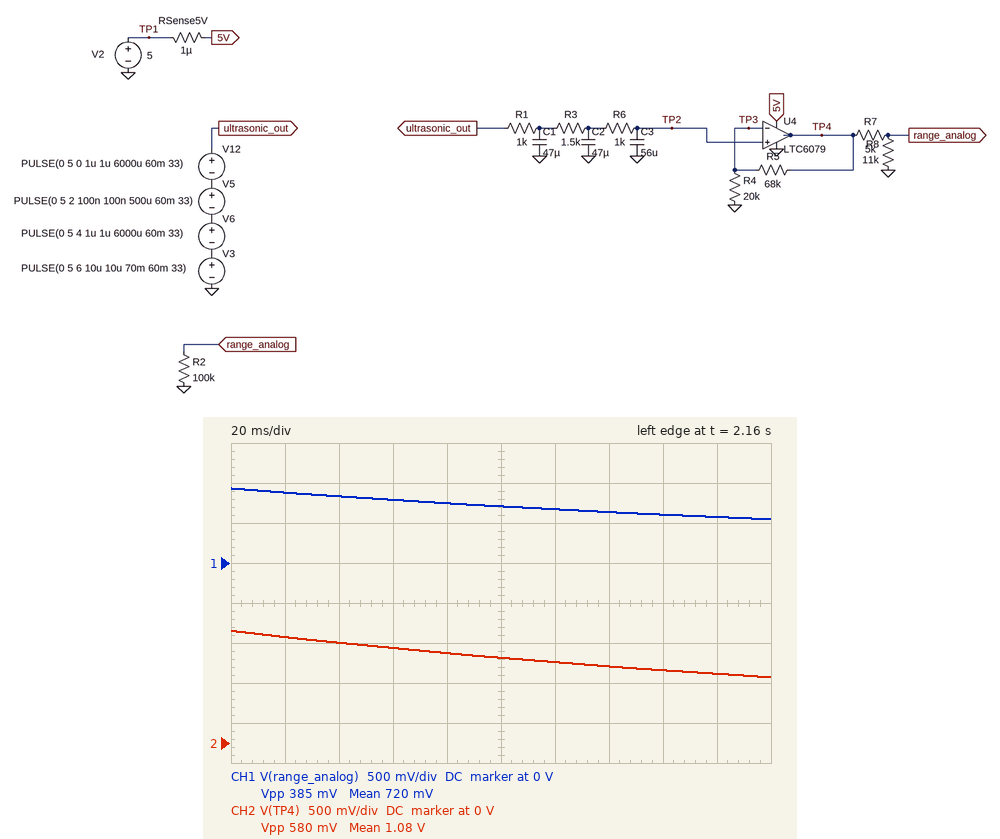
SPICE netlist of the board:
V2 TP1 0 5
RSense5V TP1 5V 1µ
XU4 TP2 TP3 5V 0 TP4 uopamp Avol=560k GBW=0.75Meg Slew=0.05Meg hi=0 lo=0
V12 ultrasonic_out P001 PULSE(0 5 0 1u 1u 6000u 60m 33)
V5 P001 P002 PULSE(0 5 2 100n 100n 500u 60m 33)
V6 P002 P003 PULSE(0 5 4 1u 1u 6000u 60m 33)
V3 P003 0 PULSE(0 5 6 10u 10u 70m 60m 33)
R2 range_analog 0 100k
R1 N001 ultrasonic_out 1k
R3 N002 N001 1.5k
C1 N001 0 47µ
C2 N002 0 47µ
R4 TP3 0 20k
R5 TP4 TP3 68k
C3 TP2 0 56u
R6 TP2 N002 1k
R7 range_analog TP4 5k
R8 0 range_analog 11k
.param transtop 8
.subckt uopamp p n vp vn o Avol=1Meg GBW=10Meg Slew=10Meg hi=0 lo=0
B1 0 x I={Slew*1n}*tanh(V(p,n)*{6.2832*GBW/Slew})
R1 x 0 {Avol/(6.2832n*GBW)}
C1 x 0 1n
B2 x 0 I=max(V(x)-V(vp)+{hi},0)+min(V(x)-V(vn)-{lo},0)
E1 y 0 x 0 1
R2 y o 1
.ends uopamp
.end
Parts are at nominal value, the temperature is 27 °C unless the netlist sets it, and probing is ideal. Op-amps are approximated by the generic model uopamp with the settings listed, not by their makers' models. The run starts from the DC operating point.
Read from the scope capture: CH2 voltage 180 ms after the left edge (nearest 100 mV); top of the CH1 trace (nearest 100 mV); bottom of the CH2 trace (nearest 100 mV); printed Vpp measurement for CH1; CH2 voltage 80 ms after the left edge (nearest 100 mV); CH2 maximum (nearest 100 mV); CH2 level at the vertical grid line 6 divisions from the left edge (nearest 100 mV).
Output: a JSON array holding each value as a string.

["900 mV", "900 mV", "800 mV", "385 mV", "1.1 V", "1.4 V", "1.0 V"]
